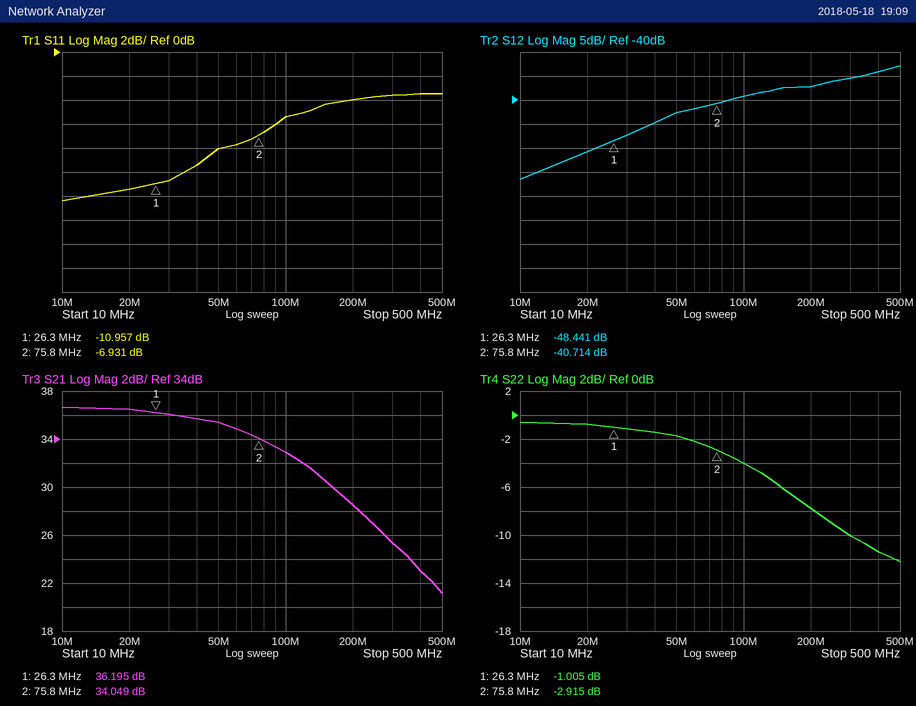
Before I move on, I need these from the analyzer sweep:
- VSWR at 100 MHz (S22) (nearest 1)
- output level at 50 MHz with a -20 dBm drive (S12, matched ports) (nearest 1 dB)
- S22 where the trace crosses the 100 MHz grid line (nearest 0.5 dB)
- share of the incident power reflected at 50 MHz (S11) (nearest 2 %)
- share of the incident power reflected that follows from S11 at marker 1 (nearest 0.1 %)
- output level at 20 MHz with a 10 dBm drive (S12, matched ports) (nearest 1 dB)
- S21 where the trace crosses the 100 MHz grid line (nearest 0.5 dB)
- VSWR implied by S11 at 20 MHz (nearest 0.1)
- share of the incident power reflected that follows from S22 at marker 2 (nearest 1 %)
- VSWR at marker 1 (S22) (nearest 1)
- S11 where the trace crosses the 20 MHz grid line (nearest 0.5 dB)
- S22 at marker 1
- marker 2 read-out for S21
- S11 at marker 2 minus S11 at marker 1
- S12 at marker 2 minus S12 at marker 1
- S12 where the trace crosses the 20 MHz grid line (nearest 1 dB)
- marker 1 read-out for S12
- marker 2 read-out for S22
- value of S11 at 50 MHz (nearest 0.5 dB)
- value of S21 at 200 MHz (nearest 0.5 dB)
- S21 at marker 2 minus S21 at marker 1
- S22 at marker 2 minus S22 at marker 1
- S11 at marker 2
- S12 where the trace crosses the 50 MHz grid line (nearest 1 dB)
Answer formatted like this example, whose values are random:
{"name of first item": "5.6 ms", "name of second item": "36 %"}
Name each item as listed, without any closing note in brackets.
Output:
{"VSWR at 100 MHz (S22)": "4", "output level at 50 MHz with a -20 dBm drive (S12, matched ports)": "-63 dBm", "S22 where the trace crosses the 100 MHz grid line": "-4.0 dB", "share of the incident power reflected at 50 MHz (S11)": "16 %", "share of the incident power reflected that follows from S11 at marker 1": "8.0 %", "output level at 20 MHz with a 10 dBm drive (S12, matched ports)": "-41 dBm", "S21 where the trace crosses the 100 MHz grid line": "33.0 dB", "VSWR implied by S11 at 20 MHz": "1.7", "share of the incident power reflected that follows from S22 at marker 2": "51 %", "VSWR at marker 1 (S22)": "17", "S11 where the trace crosses the 20 MHz grid line": "-11.5 dB", "S22 at marker 1": "-1.005 dB", "marker 2 read-out for S21": "34.049 dB", "S11 at marker 2 minus S11 at marker 1": "4.026 dB", "S12 at marker 2 minus S12 at marker 1": "7.727 dB", "S12 where the trace crosses the 20 MHz grid line": "-51 dB", "marker 1 read-out for S12": "-48.441 dB", "marker 2 read-out for S22": "-2.915 dB", "value of S11 at 50 MHz": "-8.0 dB", "value of S21 at 200 MHz": "28.5 dB", "S21 at marker 2 minus S21 at marker 1": "-2.146 dB", "S22 at marker 2 minus S22 at marker 1": "-1.910 dB", "S11 at marker 2": "-6.931 dB", "S12 where the trace crosses the 50 MHz grid line": "-43 dB"}
